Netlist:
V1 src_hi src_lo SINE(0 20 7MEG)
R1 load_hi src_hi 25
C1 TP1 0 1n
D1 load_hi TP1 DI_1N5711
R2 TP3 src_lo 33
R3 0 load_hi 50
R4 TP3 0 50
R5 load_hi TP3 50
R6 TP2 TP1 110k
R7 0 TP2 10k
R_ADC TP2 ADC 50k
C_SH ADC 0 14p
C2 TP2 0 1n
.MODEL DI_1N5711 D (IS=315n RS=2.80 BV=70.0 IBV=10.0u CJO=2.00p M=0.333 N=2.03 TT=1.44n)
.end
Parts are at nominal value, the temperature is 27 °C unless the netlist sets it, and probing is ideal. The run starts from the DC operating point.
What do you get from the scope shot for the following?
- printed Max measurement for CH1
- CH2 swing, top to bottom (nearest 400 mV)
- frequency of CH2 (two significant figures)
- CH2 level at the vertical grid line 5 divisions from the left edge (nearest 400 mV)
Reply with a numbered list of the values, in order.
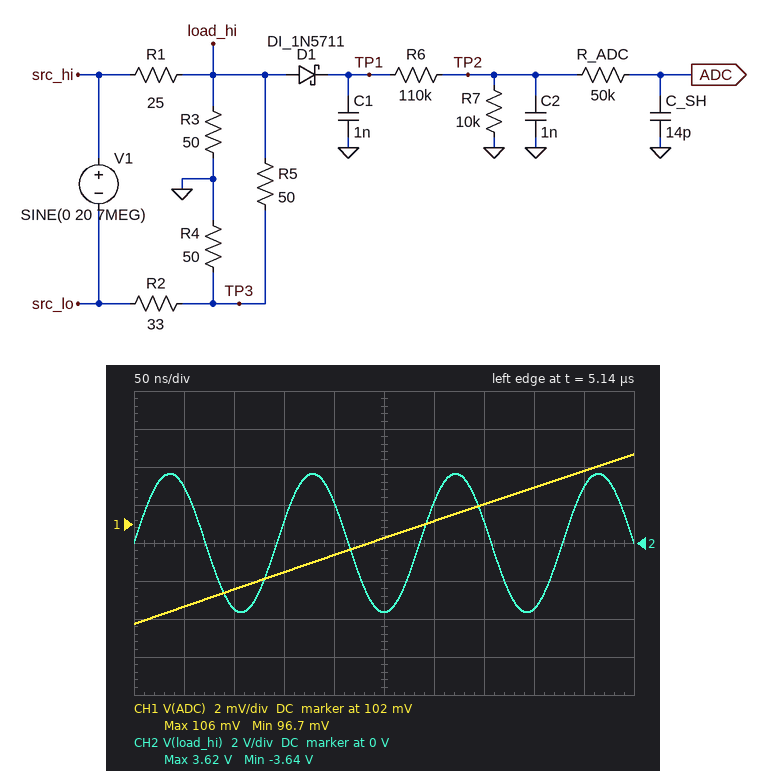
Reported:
1. 106 mV
2. 7.2 V
3. 7.0 MHz
4. -3.6 V
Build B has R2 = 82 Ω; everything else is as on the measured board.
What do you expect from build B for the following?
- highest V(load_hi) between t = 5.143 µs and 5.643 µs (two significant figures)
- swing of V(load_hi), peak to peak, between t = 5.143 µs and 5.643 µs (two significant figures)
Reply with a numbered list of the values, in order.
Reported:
1. 2.4 V
2. 4.7 V
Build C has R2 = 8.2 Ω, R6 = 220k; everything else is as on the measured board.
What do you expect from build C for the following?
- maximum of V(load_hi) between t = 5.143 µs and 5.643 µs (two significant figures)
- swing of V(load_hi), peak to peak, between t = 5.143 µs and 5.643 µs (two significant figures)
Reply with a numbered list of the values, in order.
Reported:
1. 5.0 V
2. 10 V
